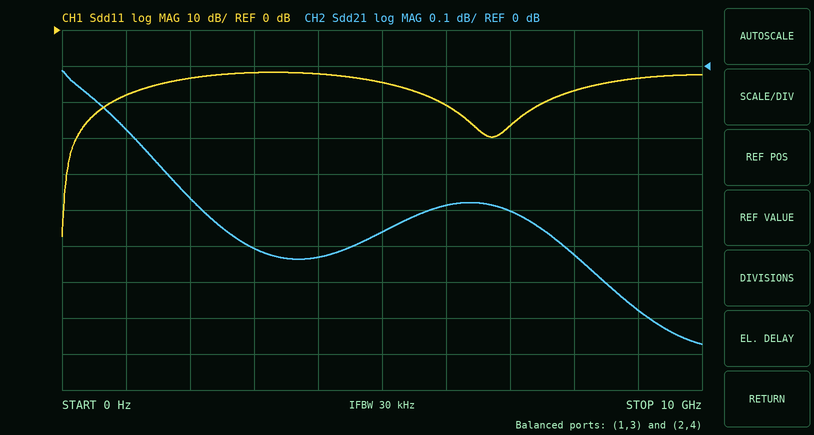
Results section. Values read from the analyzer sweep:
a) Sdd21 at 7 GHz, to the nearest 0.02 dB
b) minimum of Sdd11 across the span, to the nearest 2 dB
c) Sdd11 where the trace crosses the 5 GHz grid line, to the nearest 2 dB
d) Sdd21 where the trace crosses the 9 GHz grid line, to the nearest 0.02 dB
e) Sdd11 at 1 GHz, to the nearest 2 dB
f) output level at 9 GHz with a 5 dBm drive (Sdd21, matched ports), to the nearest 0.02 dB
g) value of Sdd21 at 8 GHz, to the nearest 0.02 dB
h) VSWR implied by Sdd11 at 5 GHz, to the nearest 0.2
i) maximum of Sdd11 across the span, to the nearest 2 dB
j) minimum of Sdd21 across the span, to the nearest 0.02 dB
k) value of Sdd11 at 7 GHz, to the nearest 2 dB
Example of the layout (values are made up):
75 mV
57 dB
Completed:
-0.40 dB
-58 dB
-14 dB
-0.68 dB
-18 dB
4.32 dBm
-0.52 dB
1.4
-12 dB
-0.78 dB
-26 dB
